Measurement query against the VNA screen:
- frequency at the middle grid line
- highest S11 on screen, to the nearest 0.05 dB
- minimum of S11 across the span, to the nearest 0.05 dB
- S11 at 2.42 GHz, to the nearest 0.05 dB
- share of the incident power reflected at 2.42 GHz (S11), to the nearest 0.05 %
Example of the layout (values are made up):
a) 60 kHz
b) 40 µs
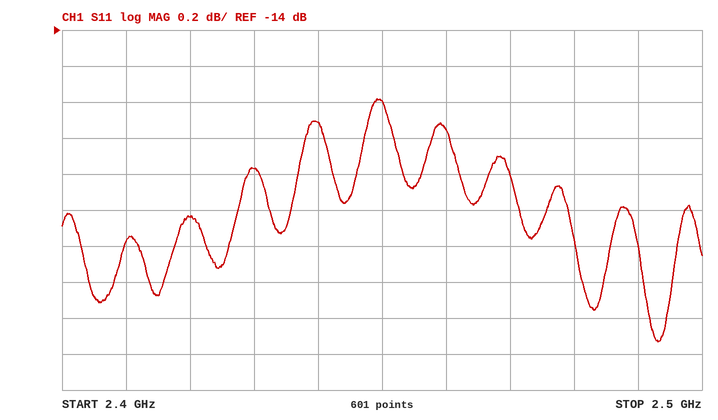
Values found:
a) 2.45 GHz
b) -14.40 dB
c) -15.75 dB
d) -15.05 dB
e) 3.15 %
